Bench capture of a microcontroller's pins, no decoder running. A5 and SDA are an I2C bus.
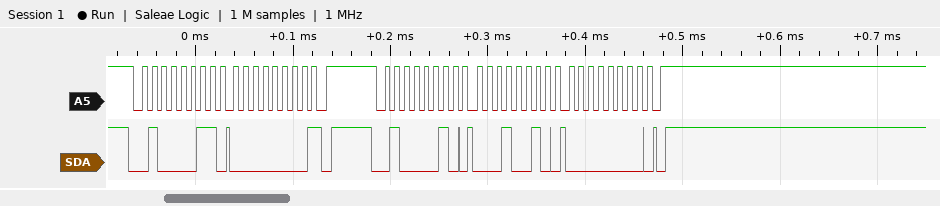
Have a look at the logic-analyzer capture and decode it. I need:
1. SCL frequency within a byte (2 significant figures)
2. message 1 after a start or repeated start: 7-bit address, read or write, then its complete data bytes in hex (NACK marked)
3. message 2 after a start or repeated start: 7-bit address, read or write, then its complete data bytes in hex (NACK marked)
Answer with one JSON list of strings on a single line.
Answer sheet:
["100 kHz", "0x21 read: 00 NACK", "0x21 write: 12 00"]
